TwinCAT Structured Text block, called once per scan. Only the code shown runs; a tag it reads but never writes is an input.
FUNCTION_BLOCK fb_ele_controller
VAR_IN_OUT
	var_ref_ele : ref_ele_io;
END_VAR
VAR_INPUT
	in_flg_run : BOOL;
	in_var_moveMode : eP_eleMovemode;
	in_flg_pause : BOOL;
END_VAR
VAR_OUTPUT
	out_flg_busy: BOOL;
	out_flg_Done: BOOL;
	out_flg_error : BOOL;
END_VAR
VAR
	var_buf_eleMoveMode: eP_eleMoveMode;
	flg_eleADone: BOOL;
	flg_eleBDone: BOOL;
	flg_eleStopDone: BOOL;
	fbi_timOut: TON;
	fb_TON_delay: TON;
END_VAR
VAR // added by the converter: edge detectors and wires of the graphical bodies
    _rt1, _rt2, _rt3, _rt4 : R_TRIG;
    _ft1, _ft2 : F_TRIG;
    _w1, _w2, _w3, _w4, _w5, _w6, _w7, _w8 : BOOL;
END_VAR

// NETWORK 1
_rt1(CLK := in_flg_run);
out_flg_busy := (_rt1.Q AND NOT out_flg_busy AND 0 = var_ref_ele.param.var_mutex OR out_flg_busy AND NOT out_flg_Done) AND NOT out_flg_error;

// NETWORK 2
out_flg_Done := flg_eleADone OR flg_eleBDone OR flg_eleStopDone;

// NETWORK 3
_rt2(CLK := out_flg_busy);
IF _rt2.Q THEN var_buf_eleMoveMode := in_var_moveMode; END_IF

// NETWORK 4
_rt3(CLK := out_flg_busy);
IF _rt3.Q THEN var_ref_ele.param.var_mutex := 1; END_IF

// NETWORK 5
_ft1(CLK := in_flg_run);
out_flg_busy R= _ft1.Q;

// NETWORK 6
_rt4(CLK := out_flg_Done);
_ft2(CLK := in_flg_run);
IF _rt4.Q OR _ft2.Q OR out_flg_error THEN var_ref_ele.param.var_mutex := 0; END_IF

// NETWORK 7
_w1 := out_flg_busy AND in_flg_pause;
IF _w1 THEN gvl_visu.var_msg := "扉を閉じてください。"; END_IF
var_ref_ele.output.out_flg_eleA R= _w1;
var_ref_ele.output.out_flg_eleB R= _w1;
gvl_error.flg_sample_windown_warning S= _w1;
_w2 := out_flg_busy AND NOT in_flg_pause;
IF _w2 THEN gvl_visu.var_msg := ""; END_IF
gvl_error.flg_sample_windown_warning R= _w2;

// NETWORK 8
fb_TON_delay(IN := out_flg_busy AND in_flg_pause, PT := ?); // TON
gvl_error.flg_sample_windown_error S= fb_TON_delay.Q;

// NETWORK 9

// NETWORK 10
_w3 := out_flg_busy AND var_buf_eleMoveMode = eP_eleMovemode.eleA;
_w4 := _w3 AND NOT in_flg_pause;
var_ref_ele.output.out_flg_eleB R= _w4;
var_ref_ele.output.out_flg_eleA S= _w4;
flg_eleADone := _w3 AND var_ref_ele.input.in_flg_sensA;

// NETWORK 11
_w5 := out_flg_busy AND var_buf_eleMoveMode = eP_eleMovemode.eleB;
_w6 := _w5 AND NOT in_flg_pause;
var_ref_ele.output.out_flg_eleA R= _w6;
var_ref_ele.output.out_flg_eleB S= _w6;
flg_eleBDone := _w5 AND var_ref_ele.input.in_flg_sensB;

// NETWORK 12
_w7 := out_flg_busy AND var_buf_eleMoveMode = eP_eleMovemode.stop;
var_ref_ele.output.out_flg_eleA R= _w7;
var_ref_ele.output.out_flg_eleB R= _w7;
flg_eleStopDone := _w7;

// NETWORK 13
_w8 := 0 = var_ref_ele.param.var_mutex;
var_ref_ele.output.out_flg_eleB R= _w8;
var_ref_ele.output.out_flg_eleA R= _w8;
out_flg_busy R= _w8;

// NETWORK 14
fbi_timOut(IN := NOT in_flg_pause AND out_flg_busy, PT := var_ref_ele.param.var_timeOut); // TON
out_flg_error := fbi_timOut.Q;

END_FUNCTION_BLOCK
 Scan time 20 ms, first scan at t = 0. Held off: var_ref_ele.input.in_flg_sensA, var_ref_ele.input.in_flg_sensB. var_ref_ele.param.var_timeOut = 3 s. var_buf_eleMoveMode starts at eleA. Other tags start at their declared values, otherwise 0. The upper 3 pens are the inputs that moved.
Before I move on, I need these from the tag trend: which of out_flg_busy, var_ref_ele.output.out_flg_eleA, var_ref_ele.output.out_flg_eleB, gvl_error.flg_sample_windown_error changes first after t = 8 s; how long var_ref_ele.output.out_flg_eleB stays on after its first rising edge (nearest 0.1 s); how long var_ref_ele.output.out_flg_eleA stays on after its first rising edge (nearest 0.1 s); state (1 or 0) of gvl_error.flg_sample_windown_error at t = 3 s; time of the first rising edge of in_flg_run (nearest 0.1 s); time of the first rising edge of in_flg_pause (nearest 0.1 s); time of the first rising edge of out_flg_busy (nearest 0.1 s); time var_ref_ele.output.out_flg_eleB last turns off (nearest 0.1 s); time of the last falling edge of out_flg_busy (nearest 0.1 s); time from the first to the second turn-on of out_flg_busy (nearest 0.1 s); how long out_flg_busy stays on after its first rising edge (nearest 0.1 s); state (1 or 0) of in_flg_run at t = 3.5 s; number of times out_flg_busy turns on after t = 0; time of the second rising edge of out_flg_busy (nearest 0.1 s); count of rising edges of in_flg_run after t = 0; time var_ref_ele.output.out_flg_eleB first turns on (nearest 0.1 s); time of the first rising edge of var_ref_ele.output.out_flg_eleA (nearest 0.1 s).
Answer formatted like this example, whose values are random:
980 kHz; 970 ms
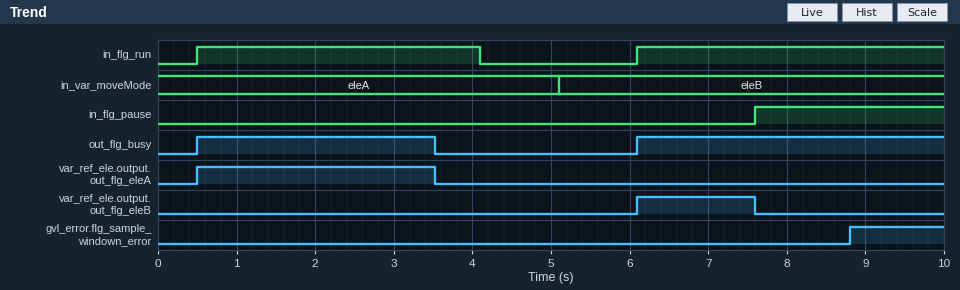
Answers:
gvl_error.flg_sample_windown_error; 1.5 s; 3.0 s; 0; 0.5 s; 7.6 s; 0.5 s; 7.6 s; 3.5 s; 5.6 s; 3.0 s; 1; 2; 6.1 s; 2; 6.1 s; 0.5 s
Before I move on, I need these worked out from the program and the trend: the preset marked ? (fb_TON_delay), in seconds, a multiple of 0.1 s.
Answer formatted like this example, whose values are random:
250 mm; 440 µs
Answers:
1.2 s
